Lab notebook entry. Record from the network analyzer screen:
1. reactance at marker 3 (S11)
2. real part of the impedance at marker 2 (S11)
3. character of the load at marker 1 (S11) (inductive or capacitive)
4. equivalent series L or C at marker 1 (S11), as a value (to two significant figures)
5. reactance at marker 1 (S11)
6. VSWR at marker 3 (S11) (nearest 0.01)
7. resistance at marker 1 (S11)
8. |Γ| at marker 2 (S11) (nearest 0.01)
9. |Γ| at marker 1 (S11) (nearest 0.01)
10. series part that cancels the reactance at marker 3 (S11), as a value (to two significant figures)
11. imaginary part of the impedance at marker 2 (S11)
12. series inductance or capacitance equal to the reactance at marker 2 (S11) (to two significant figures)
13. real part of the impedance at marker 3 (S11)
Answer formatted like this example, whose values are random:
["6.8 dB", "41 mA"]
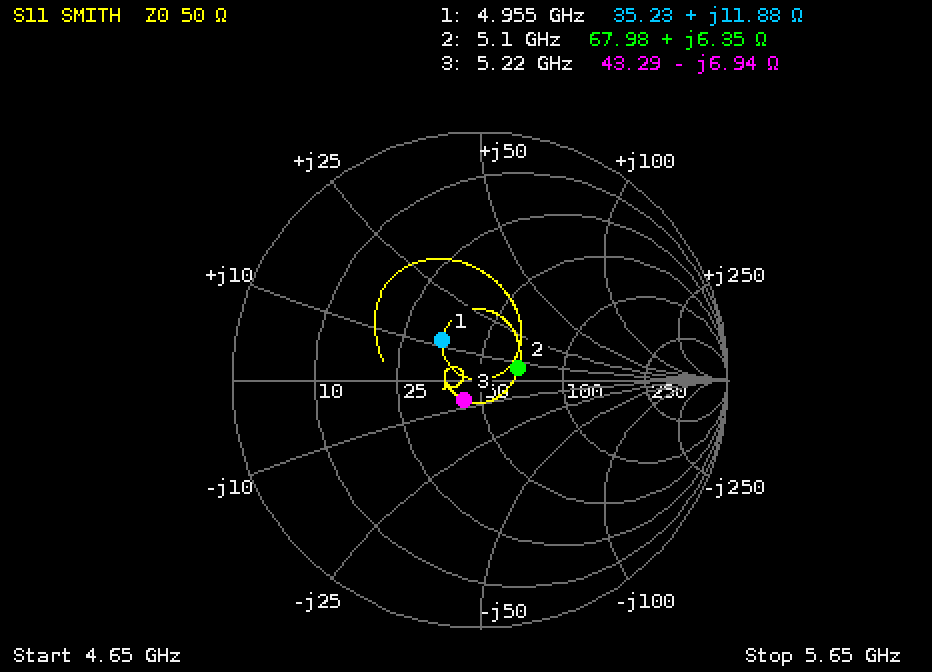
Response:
["-6.94 Ω", "67.98 Ω", "inductive", "380 pH", "+11.88 Ω", "1.23", "35.23 Ω", "0.16", "0.22", "210 pH", "+6.35 Ω", "200 pH", "43.29 Ω"]
